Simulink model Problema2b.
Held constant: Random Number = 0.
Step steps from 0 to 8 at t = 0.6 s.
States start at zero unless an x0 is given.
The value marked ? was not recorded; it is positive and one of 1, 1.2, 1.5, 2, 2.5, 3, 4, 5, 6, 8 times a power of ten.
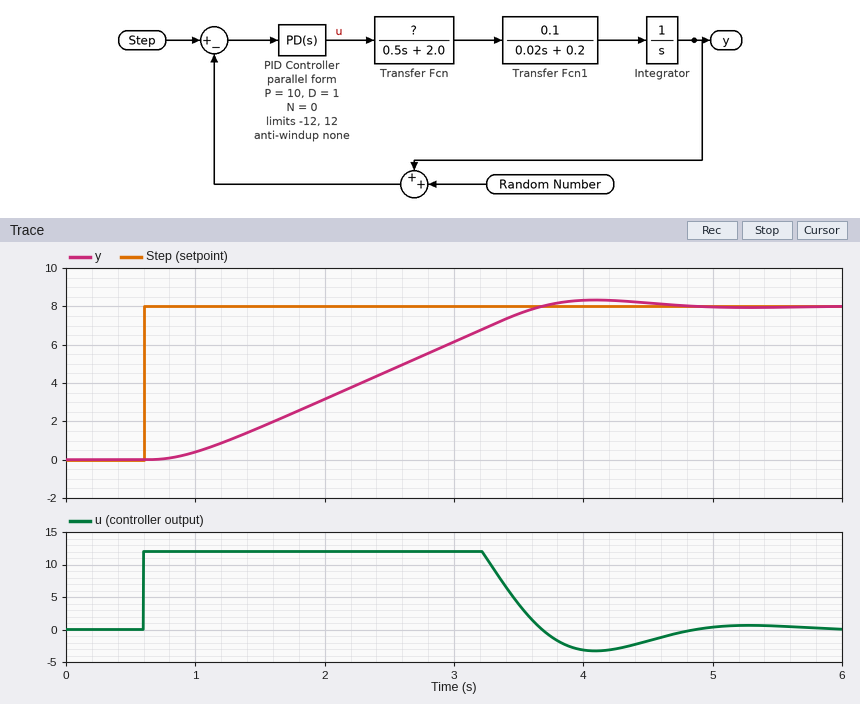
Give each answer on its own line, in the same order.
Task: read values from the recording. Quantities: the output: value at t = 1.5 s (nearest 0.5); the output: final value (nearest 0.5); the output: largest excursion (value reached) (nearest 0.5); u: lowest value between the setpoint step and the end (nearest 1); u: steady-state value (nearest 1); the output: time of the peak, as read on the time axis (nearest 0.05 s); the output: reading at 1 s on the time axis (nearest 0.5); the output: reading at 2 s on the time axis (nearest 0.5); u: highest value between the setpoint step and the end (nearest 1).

1.5
8.0
8.5
-3
0
4.10 s
0.5
3.0
12
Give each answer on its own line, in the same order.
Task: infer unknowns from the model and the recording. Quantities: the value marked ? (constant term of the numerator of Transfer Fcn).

1
